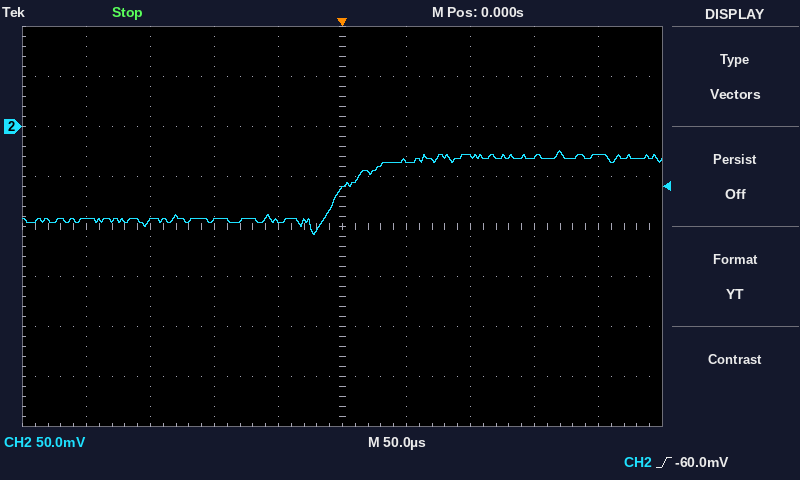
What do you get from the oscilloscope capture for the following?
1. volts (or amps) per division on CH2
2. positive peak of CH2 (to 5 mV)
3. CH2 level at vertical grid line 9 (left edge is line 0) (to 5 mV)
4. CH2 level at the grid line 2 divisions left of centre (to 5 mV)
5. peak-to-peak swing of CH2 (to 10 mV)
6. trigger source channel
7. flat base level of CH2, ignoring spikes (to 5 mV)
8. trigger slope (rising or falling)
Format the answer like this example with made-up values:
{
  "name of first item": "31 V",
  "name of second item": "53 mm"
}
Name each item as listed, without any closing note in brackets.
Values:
{
  "volts (or amps) per division on CH2": "50 mV",
  "positive peak of CH2": "-25 mV",
  "CH2 level at vertical grid line 9 (left edge is line 0)": "-30 mV",
  "CH2 level at the grid line 2 divisions left of centre": "-95 mV",
  "peak-to-peak swing of CH2": "80 mV",
  "trigger source channel": "CH2",
  "flat base level of CH2, ignoring spikes": "-90 mV",
  "trigger slope": "rising"
}
